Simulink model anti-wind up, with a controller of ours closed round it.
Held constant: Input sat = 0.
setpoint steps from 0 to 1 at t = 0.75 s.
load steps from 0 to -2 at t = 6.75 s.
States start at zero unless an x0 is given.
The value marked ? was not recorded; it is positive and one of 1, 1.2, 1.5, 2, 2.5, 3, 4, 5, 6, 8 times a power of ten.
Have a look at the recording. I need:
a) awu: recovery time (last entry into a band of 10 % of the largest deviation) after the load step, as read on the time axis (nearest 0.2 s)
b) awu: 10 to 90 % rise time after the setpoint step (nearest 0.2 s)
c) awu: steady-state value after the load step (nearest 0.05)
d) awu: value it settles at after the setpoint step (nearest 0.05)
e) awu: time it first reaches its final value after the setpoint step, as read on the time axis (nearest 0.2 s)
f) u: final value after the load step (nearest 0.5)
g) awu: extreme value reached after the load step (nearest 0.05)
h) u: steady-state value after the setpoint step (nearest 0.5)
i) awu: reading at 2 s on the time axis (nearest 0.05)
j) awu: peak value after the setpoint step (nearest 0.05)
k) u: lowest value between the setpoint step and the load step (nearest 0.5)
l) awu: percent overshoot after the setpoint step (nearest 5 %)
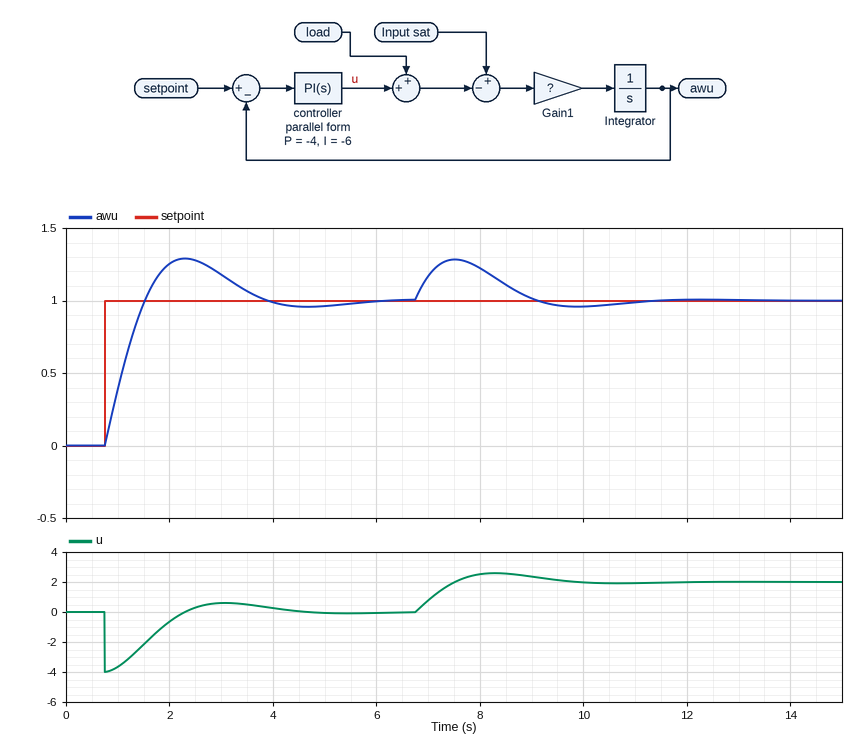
10.6 s
0.6 s
1.00
1.00
1.6 s
2.0
1.30
0.0
1.25
1.30
-4.0
30 %
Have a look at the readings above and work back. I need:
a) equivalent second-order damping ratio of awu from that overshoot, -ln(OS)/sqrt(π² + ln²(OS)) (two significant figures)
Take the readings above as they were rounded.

0.36
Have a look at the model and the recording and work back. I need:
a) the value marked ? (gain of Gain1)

0.4
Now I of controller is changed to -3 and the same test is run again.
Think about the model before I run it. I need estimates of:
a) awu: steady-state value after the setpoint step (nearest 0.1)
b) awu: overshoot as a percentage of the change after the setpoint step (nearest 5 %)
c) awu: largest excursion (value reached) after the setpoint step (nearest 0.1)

1.0
20 %
1.2
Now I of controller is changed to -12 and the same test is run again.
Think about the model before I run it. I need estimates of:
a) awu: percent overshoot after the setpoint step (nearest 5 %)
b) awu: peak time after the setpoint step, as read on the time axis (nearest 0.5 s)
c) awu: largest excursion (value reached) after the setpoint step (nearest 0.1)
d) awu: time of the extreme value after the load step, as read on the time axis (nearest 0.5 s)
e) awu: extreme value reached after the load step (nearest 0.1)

40 %
2.0 s
1.4
7.5 s
1.2
